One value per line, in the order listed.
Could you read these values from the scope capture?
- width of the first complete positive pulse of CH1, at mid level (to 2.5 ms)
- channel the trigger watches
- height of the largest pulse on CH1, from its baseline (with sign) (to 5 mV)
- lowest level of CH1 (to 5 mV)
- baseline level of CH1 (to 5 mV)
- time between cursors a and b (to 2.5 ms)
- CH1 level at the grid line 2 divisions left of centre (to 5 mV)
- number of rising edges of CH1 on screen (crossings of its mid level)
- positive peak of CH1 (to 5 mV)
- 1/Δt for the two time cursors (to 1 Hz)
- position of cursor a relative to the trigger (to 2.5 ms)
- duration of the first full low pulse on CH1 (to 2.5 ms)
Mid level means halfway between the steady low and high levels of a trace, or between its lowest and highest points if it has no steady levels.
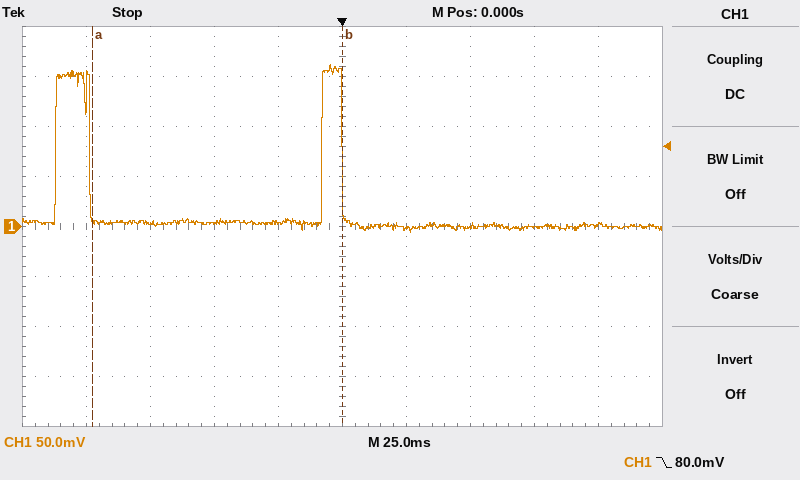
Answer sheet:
12.5 ms
CH1
+160 mV
-5 mV
0 mV
97.5 ms
5 mV
2
160 mV
10 Hz
-97.5 ms
90.0 ms
